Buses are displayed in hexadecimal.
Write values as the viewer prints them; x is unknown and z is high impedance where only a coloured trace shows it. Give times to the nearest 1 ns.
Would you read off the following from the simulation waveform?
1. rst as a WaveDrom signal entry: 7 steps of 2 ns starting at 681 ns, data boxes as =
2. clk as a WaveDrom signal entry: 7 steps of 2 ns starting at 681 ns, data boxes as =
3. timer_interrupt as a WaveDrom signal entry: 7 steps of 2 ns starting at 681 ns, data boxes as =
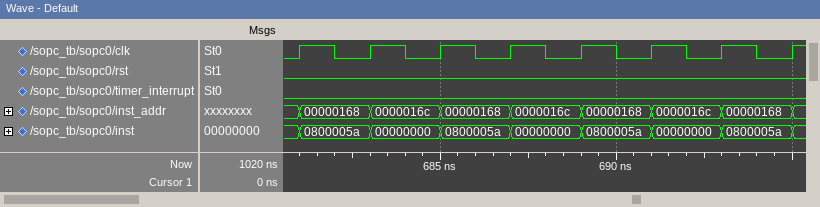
{name: 'rst', wave: '0......'}
{name: 'clk', wave: 'p......'}
{name: 'timer_interrupt', wave: '0......'}
